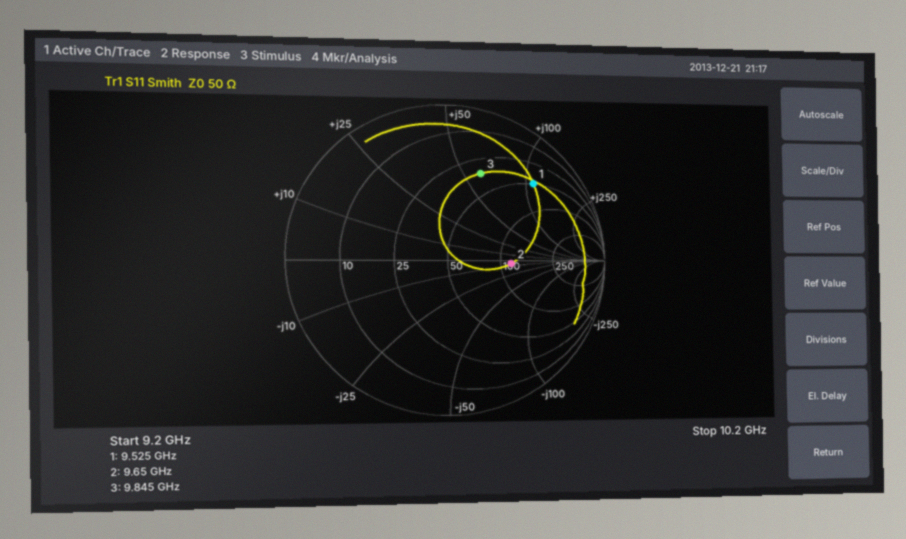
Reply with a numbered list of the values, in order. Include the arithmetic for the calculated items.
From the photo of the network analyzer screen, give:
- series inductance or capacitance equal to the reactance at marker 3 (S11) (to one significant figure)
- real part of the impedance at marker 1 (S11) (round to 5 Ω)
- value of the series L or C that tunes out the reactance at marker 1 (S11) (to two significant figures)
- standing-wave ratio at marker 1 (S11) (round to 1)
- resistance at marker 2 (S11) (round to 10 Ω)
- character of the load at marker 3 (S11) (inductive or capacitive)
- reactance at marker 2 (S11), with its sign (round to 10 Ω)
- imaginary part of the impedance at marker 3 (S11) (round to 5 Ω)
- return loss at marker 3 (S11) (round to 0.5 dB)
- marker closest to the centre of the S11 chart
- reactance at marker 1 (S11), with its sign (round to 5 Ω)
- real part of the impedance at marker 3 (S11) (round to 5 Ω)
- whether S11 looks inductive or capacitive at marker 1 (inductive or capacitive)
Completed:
1. L = 60 Ω/(2π × 9.845 GHz) ≈ 1.0 nH
2. 50 Ω
3. C = 1/(2π × 9.525 GHz × 110 Ω) ≈ 152 fF, so 150 fF to two significant figures
4. 7
5. 120 Ω
6. inductive
7. -10 Ω
8. +60 Ω
9. 4.5 dB
10. marker 2
11. +110 Ω
12. 35 Ω
13. inductive
